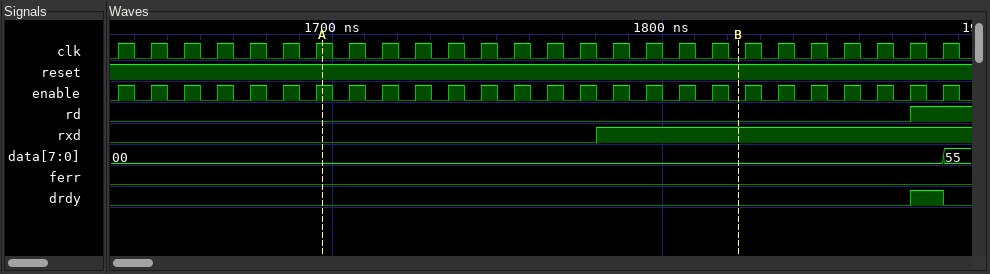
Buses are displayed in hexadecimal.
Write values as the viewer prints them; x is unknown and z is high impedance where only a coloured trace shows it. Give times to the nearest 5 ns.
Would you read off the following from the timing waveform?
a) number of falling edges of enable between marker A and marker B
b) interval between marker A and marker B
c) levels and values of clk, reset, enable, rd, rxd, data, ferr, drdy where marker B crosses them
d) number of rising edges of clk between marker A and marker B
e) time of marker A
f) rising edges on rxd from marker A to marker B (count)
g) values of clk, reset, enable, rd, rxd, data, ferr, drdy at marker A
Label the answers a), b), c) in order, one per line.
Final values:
a) 13
b) 125 ns
c) clk=0, reset=1, enable=0, rd=0, rxd=1, data=00, ferr=0, drdy=0
d) 12
e) 1695 ns
f) 1
g) clk=1, reset=1, enable=1, rd=0, rxd=0, data=00, ferr=0, drdy=0
